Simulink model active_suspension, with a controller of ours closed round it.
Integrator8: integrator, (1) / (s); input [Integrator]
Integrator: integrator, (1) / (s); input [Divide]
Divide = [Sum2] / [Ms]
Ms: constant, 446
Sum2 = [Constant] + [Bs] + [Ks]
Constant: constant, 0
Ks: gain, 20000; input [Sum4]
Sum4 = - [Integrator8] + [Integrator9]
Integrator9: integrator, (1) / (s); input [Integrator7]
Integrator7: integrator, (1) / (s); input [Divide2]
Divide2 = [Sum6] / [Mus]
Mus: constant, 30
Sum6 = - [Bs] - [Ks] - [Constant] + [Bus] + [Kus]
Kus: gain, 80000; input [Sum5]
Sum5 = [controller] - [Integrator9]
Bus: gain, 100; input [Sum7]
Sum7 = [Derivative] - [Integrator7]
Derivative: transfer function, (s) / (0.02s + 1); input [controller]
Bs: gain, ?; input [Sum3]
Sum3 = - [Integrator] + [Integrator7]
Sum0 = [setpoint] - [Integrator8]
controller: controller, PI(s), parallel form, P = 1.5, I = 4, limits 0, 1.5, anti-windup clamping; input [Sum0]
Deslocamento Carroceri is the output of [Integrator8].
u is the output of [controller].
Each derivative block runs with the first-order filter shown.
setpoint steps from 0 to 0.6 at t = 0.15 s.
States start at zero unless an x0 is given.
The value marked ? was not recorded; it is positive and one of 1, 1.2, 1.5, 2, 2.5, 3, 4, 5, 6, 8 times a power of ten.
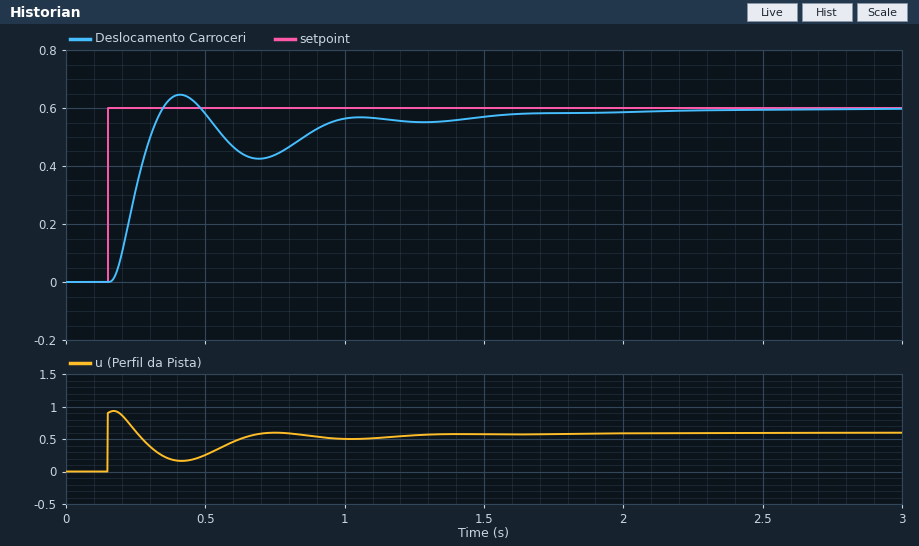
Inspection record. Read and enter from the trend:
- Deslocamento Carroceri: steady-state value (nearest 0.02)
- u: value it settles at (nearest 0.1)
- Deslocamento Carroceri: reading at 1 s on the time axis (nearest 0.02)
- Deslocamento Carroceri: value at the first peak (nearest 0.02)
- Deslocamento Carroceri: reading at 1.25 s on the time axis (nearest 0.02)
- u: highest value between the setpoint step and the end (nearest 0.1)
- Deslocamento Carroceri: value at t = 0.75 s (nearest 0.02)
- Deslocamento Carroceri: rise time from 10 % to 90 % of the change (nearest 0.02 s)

0.60
0.6
0.56
0.64
0.56
0.9
0.44
0.12 s
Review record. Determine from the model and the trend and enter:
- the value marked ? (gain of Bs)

2000
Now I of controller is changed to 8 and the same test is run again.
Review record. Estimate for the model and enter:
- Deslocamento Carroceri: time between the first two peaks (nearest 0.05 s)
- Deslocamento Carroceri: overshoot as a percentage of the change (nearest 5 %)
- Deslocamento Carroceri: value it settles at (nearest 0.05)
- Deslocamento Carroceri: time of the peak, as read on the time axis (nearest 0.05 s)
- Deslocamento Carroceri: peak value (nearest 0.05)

0.60 s
25 %
0.60
0.40 s
0.75
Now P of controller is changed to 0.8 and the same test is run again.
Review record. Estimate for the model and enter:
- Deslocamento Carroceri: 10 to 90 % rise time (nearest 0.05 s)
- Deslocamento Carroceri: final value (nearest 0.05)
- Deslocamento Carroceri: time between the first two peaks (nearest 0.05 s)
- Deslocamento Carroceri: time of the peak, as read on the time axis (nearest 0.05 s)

0.20 s
0.60
0.70 s
0.50 s
